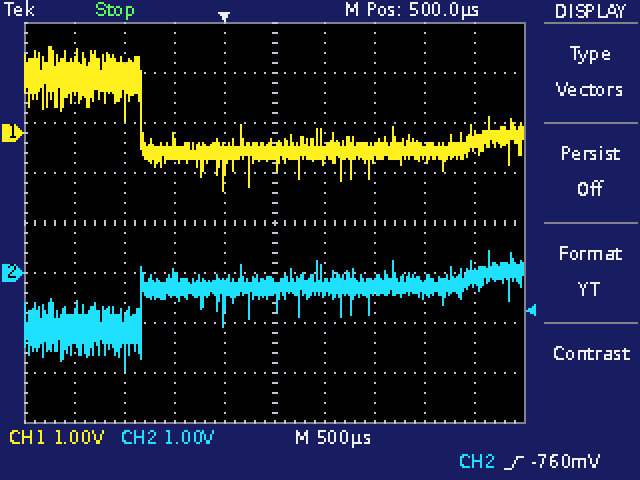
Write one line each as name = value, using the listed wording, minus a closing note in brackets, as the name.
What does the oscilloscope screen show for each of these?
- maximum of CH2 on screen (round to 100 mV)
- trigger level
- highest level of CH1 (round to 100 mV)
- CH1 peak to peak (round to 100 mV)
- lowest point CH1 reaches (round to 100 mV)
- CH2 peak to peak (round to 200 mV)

maximum of CH2 on screen = 400 mV
trigger level = -760 mV
highest level of CH1 = 1.7 V
CH1 peak to peak = 2.9 V
lowest point CH1 reaches = -1.2 V
CH2 peak to peak = 2.4 V
